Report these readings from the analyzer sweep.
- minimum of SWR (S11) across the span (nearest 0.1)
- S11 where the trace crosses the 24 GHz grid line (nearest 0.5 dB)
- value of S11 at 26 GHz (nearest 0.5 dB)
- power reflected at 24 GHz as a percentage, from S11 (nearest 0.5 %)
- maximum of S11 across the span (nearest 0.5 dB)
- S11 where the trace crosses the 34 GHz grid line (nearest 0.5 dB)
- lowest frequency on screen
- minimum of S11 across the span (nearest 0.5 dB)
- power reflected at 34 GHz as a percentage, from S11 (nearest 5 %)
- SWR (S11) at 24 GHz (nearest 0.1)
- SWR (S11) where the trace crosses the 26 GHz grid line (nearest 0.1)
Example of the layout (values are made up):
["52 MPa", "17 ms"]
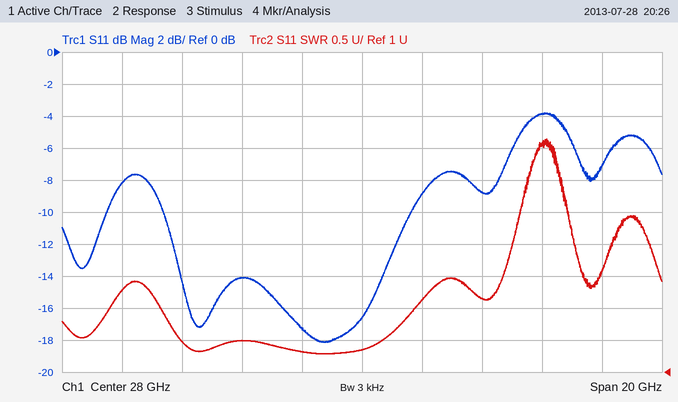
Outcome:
["1.3", "-14.0 dB", "-17.5 dB", "4.0 %", "-4.0 dB", "-4.0 dB", "18 GHz", "-18.0 dB", "40 %", "1.5", "1.3"]
